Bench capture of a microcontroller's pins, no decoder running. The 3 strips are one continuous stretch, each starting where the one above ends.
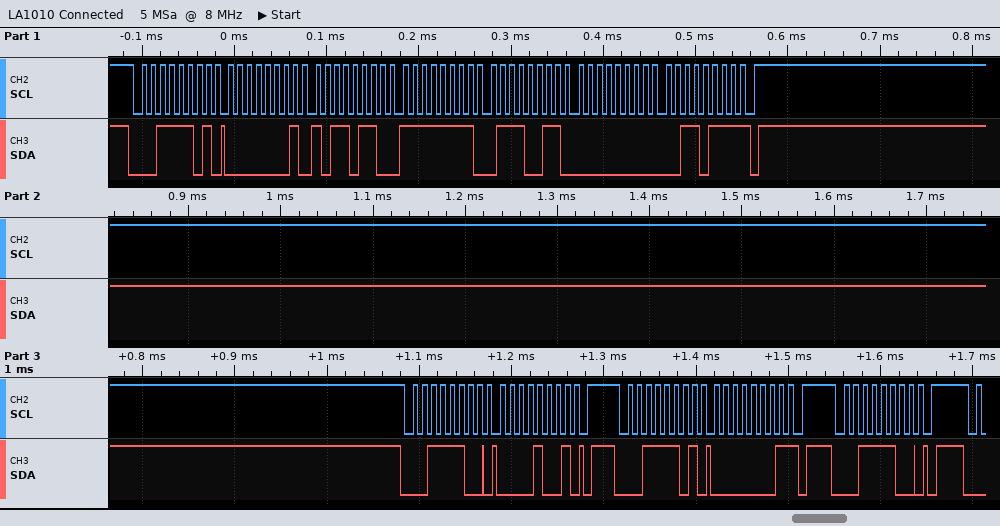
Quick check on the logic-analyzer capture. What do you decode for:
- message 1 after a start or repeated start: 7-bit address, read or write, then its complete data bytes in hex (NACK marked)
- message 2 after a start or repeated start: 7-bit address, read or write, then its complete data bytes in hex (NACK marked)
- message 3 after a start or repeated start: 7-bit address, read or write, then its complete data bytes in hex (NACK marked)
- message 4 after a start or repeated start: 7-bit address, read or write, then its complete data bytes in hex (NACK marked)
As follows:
0x1E read: 01 B6 FF 73 00 37 NACK
0x1E write: 09
0x1E read: 01 NACK
0x1E write
